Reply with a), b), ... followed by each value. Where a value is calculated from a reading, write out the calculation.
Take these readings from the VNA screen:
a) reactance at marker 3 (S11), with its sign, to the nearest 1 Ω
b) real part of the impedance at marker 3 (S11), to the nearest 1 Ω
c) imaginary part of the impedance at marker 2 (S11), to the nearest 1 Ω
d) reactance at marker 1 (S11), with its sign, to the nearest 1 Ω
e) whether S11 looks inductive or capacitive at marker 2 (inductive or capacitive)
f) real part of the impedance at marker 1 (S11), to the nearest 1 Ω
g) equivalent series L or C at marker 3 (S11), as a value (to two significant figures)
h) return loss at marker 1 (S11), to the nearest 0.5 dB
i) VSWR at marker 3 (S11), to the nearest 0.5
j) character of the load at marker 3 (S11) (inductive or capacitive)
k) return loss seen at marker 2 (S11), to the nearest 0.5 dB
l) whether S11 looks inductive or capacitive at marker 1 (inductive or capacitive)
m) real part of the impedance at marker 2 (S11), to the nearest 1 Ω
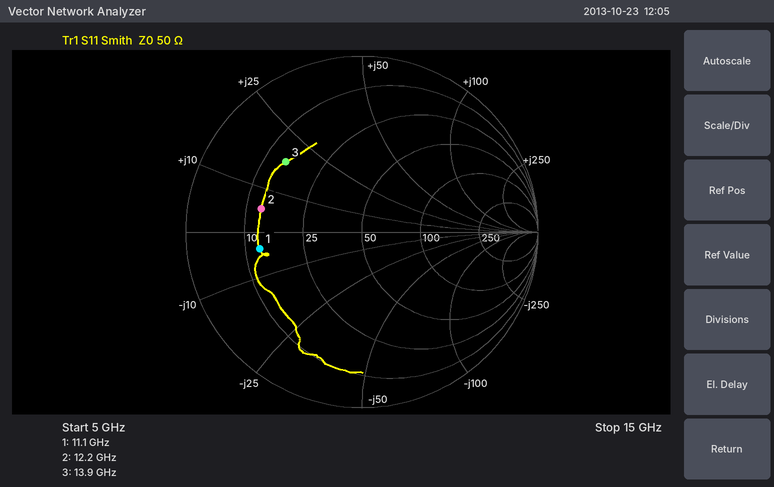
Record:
a) +18 Ω
b) 15 Ω
c) +5 Ω
d) -4 Ω
e) inductive
f) 13 Ω
g) L = 18 Ω/(2π × 13.9 GHz) ≈ 206 pH, so 210 pH to two significant figures
h) 4.5 dB
i) 4.0
j) inductive
k) 4.5 dB
l) capacitive
m) 13 Ω
